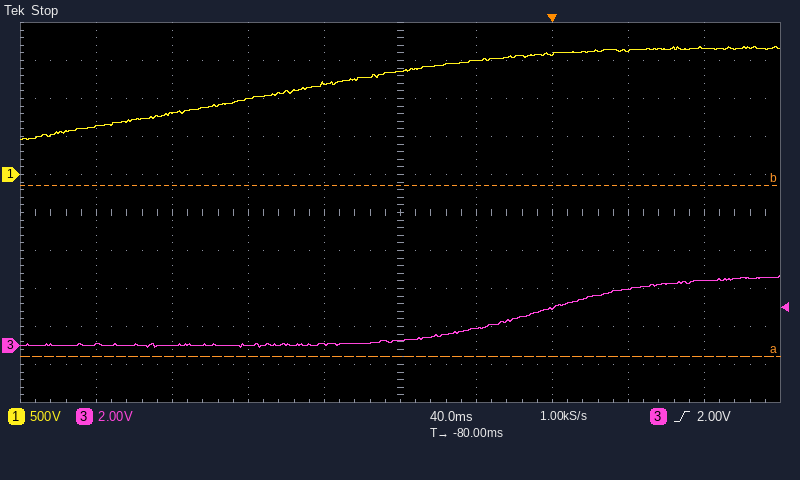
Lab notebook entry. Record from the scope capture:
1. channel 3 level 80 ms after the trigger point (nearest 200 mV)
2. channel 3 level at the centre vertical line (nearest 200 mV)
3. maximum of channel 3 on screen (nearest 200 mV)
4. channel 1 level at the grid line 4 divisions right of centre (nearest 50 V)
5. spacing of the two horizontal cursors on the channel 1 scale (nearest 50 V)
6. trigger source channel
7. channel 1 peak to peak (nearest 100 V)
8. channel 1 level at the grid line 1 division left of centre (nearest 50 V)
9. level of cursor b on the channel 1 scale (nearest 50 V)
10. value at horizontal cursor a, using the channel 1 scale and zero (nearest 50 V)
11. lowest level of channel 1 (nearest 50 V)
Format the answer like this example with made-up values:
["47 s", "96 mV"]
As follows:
["3.4 V", "200 mV", "3.6 V", "1.65 kV", "2.25 kV", "channel 3", "1.20 kV", "1.20 kV", "-150 V", "-2.40 kV", "450 V"]
